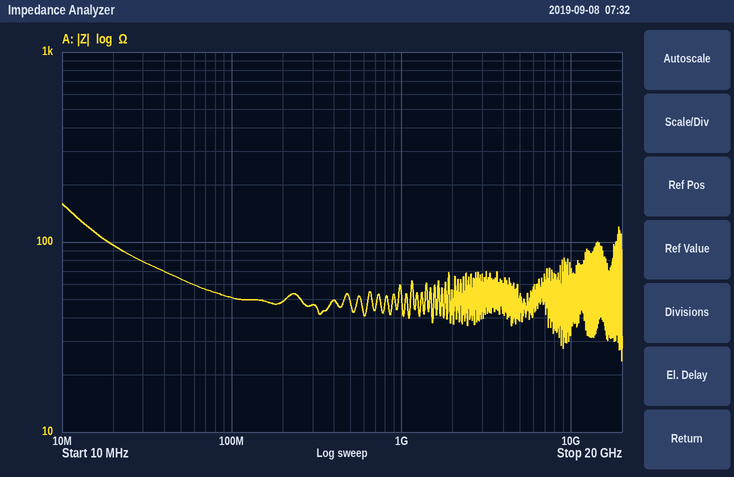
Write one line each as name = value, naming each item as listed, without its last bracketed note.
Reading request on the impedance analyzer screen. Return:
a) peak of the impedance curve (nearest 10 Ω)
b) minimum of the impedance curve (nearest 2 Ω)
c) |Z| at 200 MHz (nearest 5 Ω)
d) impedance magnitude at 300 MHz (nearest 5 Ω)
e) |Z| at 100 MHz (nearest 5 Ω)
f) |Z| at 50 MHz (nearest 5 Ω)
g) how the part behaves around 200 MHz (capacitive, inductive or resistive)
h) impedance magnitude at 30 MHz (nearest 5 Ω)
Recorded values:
peak of the impedance curve = 160 Ω
minimum of the impedance curve = 24 Ω
|Z| at 200 MHz = 50 Ω
impedance magnitude at 300 MHz = 45 Ω
|Z| at 100 MHz = 50 Ω
|Z| at 50 MHz = 65 Ω
how the part behaves around 200 MHz = resistive
impedance magnitude at 30 MHz = 80 Ω
